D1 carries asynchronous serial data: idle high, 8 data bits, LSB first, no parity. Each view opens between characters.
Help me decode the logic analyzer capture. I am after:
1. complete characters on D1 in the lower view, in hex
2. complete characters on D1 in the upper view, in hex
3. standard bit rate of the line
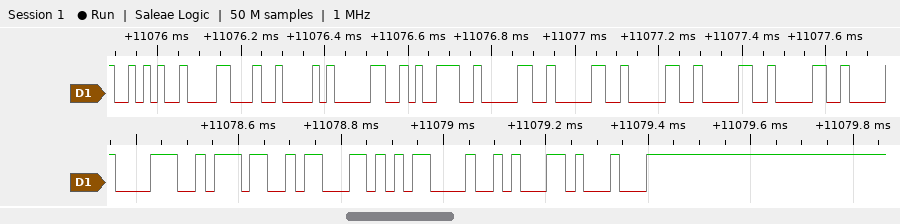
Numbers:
38, 37, 63, 0D, 8A, 11
2A, 18, 42, 30, 39, 30, 30, 30, 30, 30
57600 baud
